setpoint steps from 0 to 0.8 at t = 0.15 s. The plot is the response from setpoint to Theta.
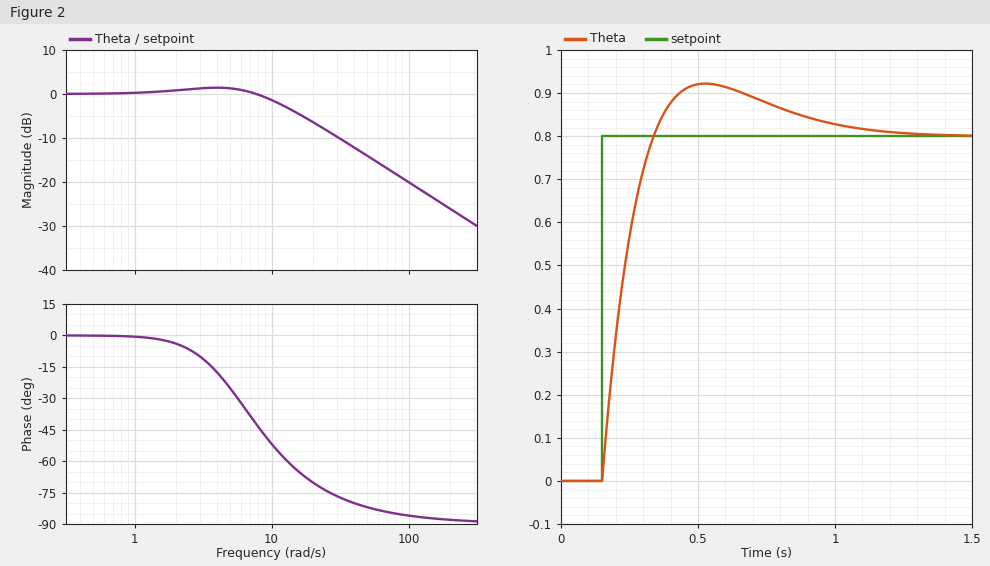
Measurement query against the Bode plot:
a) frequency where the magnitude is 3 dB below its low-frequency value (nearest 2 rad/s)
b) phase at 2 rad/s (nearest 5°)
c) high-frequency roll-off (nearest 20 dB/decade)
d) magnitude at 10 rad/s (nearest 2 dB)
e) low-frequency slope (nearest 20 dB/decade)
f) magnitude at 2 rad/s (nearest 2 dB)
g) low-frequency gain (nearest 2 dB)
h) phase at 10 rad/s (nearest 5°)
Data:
12 rad/s
-5°
-20 dB/decade
-2 dB
0 dB/decade
0 dB
0 dB
-50°
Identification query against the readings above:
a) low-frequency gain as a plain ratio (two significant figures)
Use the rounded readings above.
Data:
1.0
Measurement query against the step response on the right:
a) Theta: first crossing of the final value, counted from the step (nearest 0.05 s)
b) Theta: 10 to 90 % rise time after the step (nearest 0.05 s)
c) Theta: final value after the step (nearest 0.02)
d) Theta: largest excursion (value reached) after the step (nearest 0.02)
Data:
0.20 s
0.15 s
0.80
0.92
